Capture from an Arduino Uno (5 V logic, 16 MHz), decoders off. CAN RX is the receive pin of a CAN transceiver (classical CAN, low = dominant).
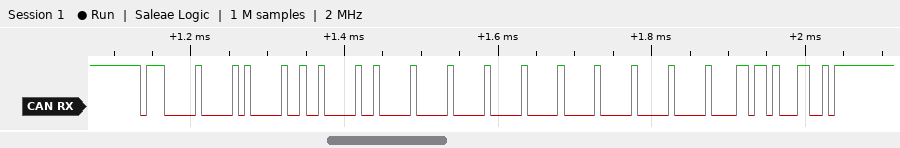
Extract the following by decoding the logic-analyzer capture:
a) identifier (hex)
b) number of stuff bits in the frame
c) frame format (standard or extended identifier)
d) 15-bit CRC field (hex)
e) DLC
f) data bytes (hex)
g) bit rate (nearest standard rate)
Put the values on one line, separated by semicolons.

0x700; 13; standard; 0x368C; 8; 09 01 00 00 00 00 00 00; 125 kbit/s
